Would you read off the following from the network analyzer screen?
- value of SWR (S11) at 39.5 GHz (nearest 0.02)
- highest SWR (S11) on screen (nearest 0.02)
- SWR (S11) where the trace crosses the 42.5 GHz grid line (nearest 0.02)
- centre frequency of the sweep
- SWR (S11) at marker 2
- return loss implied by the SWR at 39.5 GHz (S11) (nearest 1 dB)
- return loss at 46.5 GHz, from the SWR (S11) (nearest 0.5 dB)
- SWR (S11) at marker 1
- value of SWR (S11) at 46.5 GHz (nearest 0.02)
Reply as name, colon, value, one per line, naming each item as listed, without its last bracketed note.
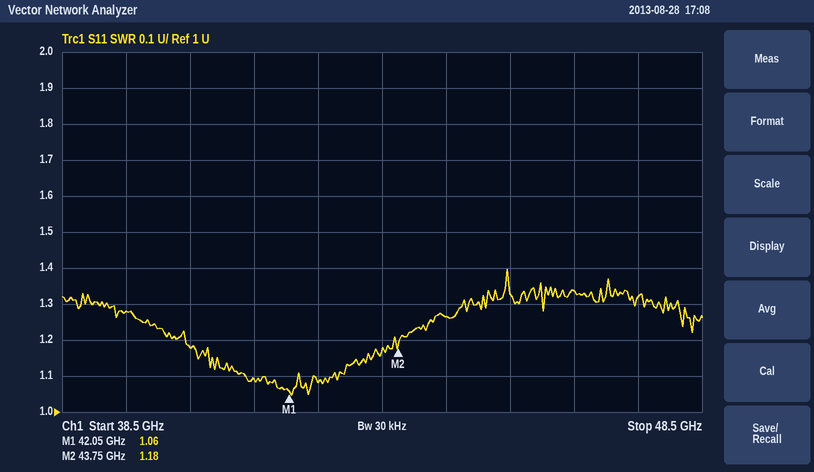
value of SWR (S11) at 39.5 GHz: 1.28
highest SWR (S11) on screen: 1.40
SWR (S11) where the trace crosses the 42.5 GHz grid line: 1.08
centre frequency of the sweep: 43.5 GHz
SWR (S11) at marker 2: 1.18
return loss implied by the SWR at 39.5 GHz (S11): 18 dB
return loss at 46.5 GHz, from the SWR (S11): 17.0 dB
SWR (S11) at marker 1: 1.06
value of SWR (S11) at 46.5 GHz: 1.34
